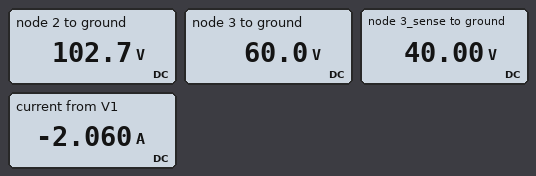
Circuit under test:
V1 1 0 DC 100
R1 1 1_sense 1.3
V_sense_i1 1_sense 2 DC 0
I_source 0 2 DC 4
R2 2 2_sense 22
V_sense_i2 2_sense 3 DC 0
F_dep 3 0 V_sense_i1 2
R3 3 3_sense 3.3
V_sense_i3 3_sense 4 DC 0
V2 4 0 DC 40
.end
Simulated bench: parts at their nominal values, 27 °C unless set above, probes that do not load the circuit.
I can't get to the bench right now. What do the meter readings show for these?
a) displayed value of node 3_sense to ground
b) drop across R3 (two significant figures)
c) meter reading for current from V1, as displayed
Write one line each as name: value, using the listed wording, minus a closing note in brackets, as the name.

displayed value of node 3_sense to ground: 40.00 V
drop across R3: 20 V
meter reading for current from V1, as displayed: -2.060 A
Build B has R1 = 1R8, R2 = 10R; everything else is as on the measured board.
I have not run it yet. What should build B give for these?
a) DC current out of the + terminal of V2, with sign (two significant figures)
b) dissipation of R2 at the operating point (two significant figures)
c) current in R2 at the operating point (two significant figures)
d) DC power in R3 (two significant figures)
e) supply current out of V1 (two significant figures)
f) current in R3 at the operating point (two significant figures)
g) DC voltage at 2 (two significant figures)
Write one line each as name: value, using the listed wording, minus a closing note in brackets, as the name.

DC current out of the + terminal of V2, with sign: -3.2 A
dissipation of R2 at the operating point: 230 W
current in R2 at the operating point: 4.8 A
DC power in R3: 34 W
supply current out of V1: 800 mA
current in R3 at the operating point: 3.2 A
DC voltage at 2: 99 V
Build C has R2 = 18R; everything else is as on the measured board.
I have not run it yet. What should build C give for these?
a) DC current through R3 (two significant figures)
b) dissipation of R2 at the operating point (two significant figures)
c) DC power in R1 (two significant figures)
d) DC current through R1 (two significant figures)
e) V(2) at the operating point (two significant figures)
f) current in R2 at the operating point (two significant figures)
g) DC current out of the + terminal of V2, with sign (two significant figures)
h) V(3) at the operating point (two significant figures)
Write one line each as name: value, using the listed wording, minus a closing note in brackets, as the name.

DC current through R3: 5.6 A
dissipation of R2 at the operating point: 110 W
DC power in R1: 3.2 W
DC current through R1: 1.6 A
V(2) at the operating point: 100 V
current in R2 at the operating point: 2.4 A
DC current out of the + terminal of V2, with sign: -5.6 A
V(3) at the operating point: 58 V
